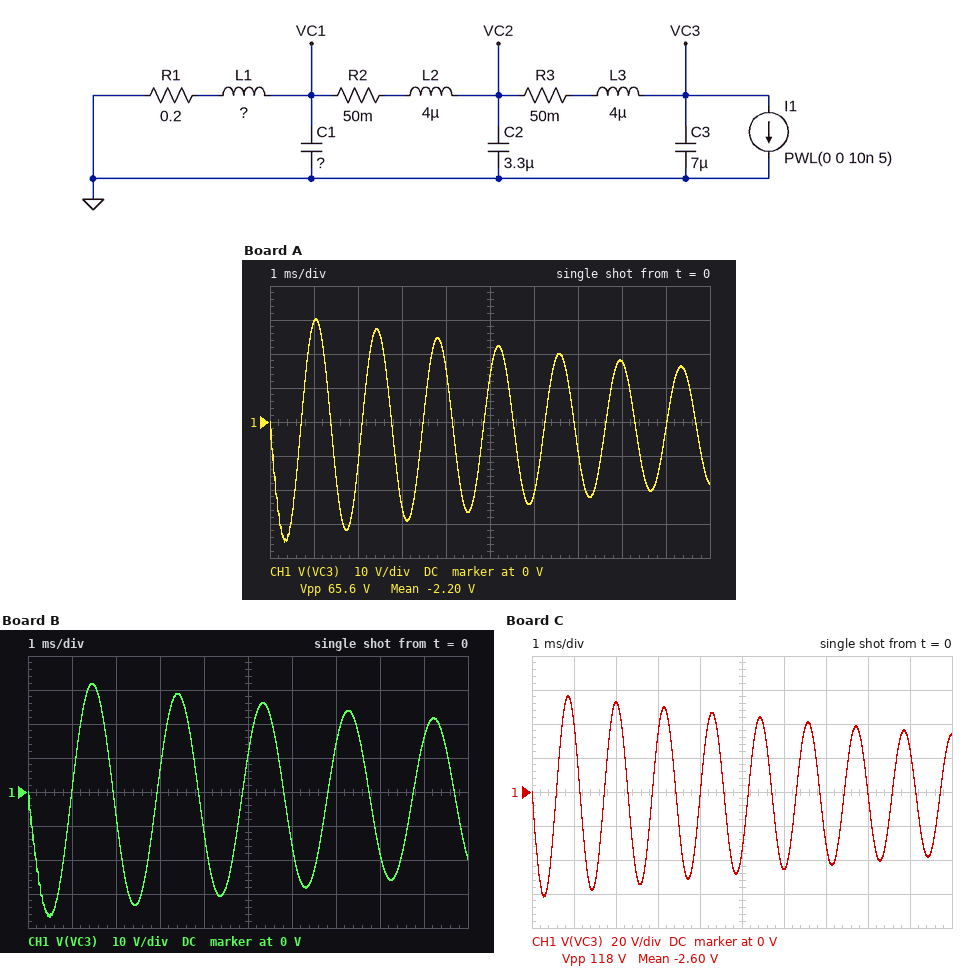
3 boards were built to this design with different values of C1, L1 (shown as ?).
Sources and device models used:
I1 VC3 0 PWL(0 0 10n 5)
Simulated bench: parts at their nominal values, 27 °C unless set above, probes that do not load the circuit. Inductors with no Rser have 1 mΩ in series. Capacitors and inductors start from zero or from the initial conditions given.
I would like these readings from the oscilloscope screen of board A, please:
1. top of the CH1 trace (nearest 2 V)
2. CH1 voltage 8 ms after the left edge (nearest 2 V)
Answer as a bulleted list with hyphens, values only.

- 30 V
- 18 V
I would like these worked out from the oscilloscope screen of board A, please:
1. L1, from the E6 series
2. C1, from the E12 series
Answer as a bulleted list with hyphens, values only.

- 1.5 mH
- 22 µF
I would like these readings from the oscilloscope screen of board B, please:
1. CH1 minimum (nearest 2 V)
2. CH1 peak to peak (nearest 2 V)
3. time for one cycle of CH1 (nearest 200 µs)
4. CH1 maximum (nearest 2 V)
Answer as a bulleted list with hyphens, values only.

- -36 V
- 68 V
- 2.0 ms
- 32 V
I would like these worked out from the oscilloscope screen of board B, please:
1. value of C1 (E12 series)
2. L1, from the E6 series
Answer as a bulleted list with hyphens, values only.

- 33 µF
- 2.2 mH
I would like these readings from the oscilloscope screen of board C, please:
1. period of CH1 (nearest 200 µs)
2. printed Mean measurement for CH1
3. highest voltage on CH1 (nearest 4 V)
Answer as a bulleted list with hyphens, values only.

- 1.2 ms
- -2.60 V
- 56 V
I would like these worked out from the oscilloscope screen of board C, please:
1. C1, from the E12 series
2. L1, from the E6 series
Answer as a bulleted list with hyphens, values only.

- 4.7 µF
- 2.2 mH
